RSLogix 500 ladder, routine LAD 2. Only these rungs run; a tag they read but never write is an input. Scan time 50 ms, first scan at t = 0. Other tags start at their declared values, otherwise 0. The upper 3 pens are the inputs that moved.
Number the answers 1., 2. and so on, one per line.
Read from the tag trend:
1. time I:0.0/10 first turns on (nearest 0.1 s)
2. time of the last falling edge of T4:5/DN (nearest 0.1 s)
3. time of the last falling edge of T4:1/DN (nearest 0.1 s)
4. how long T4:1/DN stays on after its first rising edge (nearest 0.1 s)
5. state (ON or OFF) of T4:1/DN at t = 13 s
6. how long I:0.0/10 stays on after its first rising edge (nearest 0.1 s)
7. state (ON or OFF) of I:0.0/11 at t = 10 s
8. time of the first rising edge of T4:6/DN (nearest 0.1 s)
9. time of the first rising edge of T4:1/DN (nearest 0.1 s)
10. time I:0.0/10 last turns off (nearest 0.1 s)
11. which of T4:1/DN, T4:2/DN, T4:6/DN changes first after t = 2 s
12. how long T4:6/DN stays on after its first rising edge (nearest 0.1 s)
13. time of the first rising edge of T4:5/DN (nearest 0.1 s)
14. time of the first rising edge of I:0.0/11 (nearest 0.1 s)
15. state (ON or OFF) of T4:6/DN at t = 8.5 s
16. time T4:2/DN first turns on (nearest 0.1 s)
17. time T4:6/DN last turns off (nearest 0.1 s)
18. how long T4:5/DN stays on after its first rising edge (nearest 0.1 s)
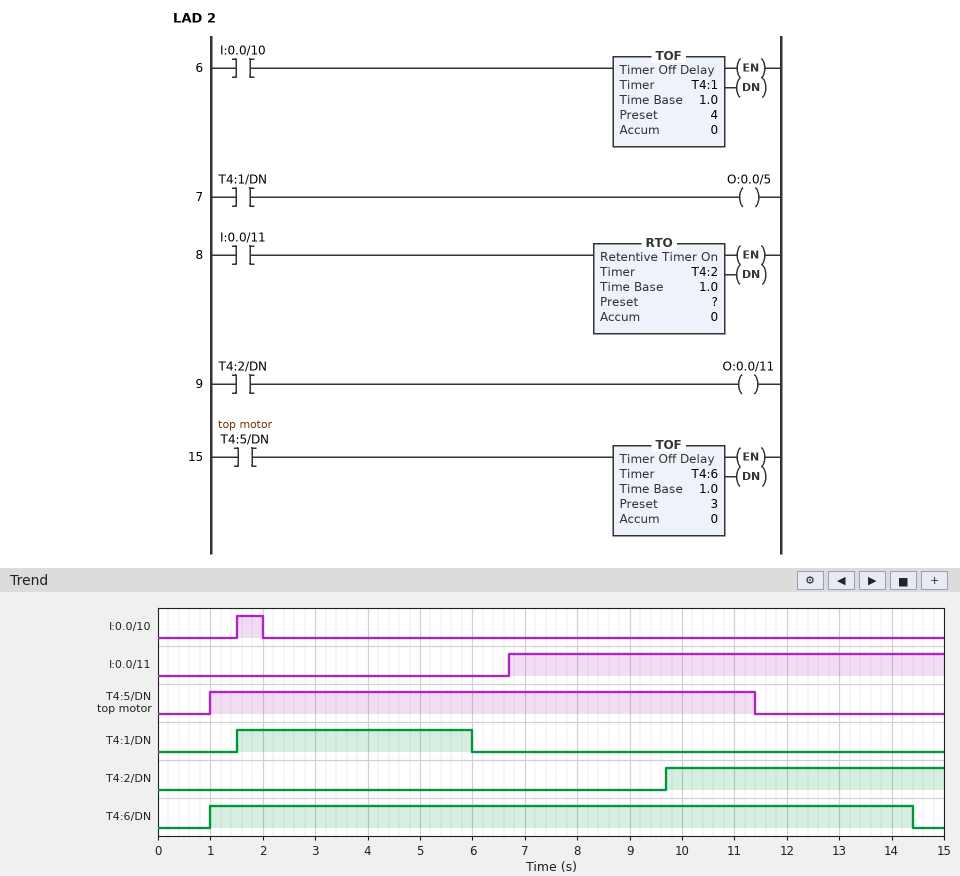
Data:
1. 1.5 s
2. 11.4 s
3. 6.0 s
4. 4.5 s
5. OFF
6. 0.5 s
7. ON
8. 1.0 s
9. 1.5 s
10. 2.0 s
11. T4:1/DN
12. 13.4 s
13. 1.0 s
14. 6.7 s
15. ON
16. 9.7 s
17. 14.4 s
18. 10.4 s
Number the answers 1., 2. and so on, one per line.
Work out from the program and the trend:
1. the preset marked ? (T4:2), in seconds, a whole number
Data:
1. 3 s
